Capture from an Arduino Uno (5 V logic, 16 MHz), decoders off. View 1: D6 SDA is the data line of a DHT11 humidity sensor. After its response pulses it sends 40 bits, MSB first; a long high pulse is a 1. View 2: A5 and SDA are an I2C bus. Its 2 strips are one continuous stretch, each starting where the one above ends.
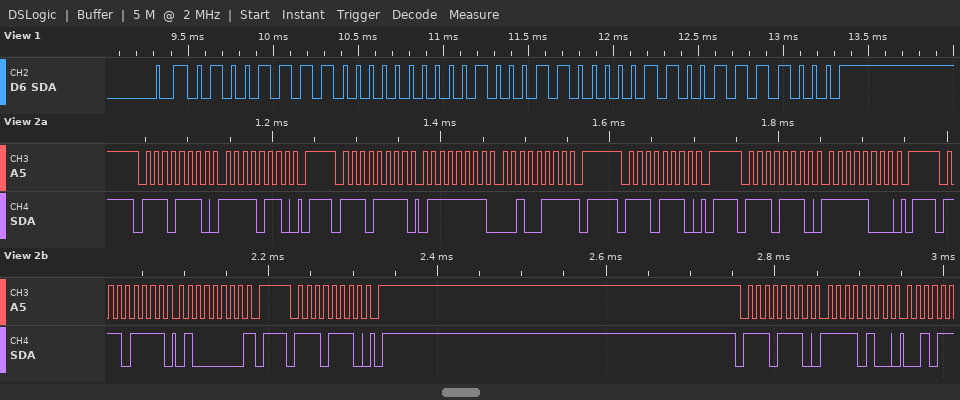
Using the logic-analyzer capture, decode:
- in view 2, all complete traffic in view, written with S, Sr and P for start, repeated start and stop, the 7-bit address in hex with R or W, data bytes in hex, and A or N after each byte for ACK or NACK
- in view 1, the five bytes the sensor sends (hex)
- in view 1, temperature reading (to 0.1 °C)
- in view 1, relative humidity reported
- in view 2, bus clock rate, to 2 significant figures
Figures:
S 77W A F6 A P S 77R A 7F A 27 N P S 77W A P S 77W A F8 A P S 77R A 40 N P S 77W A P S 77W A F4 A
4F 00 23 06 78
35.6 °C
79 %
100 kHz
